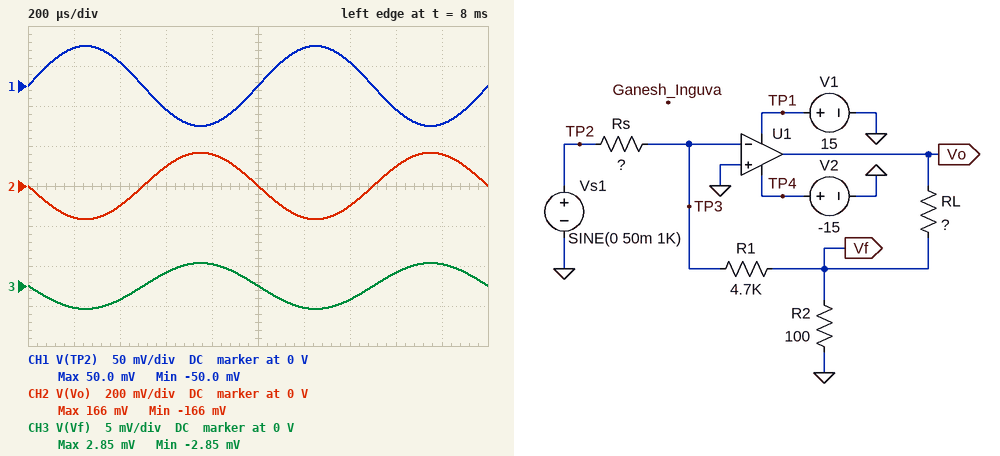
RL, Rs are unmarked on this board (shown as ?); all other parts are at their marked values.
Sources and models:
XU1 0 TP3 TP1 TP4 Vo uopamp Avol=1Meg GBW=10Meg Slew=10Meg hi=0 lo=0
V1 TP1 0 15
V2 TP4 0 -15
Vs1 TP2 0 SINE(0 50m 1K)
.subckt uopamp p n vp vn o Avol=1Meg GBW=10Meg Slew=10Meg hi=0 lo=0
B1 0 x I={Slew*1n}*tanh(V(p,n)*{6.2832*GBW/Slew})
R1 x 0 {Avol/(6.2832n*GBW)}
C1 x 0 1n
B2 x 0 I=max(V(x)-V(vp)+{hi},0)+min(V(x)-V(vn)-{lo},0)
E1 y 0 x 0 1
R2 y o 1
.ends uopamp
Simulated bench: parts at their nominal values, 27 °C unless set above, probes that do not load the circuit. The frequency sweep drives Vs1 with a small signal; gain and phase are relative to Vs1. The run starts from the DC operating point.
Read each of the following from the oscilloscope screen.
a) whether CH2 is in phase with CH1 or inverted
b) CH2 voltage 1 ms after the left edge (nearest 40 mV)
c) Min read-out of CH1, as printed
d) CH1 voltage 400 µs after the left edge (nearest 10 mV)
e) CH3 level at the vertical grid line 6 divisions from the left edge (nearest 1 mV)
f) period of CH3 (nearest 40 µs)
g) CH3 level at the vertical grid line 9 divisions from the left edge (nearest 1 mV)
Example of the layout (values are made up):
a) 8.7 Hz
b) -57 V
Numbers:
a) inverted
b) 0 V
c) -50.0 mV
d) 30 mV
e) -3 mV
f) 1.00 ms
g) 3 mV
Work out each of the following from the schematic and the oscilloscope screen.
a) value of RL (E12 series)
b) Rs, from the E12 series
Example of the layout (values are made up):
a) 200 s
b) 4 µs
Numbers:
a) 5.6 kΩ
b) 82 kΩ
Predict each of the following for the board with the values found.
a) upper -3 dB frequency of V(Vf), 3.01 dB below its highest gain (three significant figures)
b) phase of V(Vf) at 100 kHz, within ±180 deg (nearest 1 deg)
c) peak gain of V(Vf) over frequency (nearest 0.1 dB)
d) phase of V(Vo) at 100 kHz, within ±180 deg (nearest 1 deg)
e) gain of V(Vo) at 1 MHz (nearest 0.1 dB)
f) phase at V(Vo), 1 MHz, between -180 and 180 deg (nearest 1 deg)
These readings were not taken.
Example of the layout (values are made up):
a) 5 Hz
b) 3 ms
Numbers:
a) 166 kHz
b) 148 deg
c) -24.8 dB
d) 149 deg
e) -5.3 dB
f) 99 deg
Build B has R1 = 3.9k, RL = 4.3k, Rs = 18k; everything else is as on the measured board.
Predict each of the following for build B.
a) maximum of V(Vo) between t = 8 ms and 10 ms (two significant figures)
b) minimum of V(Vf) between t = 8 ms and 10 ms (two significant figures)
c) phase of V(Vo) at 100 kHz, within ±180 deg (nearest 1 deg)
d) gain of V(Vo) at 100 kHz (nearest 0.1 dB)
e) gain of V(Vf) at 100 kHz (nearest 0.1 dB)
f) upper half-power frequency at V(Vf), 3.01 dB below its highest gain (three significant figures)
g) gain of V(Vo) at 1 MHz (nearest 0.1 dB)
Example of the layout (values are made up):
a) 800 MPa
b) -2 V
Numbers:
a) 490 mV
b) -11 mV
c) 152 deg
d) 18.7 dB
e) -14.4 dB
f) 186 kHz
g) 5.0 dB
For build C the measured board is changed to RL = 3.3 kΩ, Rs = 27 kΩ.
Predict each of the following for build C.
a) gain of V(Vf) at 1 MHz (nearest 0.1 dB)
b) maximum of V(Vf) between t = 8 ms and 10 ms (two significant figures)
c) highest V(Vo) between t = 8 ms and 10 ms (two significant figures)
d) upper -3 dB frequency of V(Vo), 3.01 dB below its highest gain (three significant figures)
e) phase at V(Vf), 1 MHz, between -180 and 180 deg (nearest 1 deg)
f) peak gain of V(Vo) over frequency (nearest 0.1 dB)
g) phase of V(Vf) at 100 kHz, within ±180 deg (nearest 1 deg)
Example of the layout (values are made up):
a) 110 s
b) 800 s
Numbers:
a) -27.5 dB
b) 8.7 mV
c) 300 mV
d) 250 kHz
e) 100 deg
f) 15.6 dB
g) 158 deg
